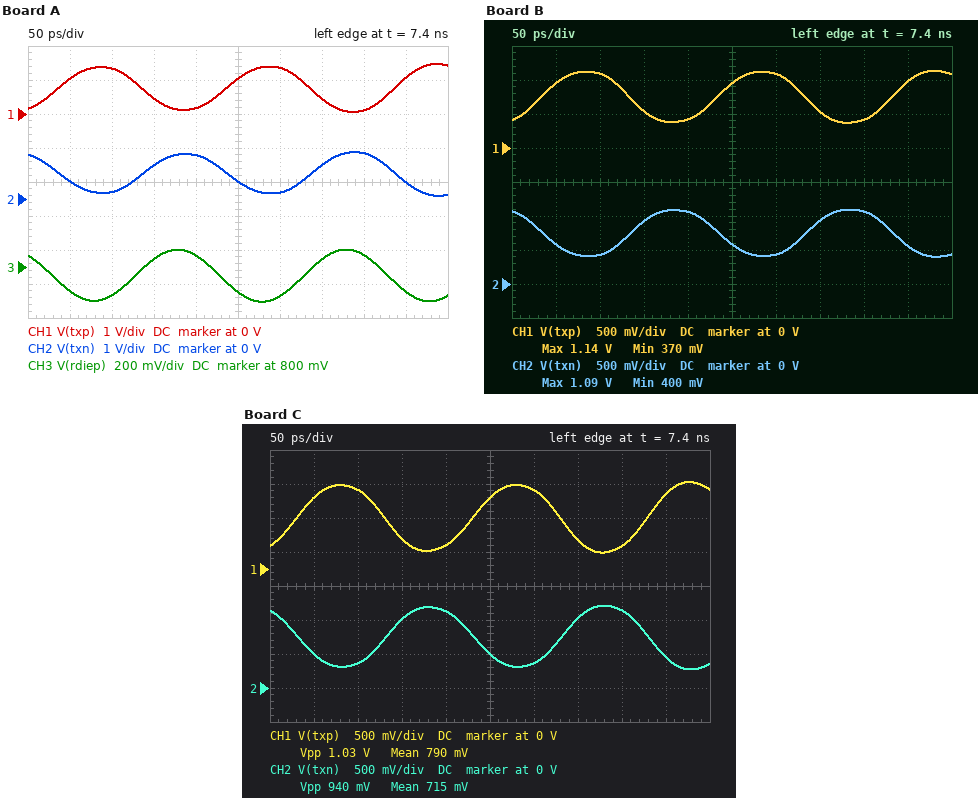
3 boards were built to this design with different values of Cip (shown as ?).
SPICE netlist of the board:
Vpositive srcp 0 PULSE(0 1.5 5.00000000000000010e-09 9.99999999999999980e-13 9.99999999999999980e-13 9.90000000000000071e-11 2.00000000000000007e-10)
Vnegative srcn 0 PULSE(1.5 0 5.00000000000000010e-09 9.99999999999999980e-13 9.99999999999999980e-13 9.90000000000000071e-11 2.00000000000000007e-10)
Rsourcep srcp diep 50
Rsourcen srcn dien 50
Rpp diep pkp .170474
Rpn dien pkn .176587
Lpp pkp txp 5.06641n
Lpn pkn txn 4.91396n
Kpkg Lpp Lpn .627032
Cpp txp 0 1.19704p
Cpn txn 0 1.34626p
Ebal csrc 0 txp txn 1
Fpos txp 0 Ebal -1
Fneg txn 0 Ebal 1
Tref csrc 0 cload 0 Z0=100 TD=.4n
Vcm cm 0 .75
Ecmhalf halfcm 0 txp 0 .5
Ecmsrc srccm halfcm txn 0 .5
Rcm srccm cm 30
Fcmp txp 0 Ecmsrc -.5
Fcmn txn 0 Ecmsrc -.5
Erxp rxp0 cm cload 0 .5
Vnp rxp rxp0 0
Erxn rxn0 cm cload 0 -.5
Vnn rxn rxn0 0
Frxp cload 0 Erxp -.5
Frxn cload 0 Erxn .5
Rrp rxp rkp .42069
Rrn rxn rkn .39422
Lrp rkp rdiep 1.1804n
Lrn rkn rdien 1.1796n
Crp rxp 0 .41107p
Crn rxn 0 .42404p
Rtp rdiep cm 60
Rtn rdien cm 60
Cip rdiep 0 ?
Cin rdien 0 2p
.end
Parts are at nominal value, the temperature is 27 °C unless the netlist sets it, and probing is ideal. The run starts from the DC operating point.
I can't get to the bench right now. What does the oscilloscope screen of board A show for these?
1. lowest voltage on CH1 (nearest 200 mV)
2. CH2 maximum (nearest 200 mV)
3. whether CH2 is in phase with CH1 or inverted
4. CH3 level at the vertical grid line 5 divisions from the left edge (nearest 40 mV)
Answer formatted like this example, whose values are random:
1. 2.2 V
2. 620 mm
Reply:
1. 0 V
2. 1.4 V
3. inverted
4. 640 mV
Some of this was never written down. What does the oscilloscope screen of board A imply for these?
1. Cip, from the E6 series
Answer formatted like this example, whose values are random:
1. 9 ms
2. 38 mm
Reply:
1. 4.7 pF
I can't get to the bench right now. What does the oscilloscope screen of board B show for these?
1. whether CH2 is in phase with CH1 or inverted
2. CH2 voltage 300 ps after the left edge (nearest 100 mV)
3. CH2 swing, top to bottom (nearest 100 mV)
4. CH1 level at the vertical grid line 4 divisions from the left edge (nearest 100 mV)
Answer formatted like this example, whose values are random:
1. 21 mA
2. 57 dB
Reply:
1. inverted
2. 400 mV
3. 700 mV
4. 400 mV
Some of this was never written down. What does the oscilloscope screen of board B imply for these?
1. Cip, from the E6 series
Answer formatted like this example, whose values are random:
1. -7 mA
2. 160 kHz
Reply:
1. 1 pF
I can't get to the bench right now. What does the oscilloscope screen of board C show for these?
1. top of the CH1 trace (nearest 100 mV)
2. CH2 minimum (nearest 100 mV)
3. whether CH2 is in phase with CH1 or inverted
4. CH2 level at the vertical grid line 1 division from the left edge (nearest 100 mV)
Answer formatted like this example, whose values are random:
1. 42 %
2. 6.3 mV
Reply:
1. 1.3 V
2. 300 mV
3. inverted
4. 500 mV
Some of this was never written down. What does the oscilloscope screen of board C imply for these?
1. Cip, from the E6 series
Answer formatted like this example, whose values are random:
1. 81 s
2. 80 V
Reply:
1. 1.5 pF
